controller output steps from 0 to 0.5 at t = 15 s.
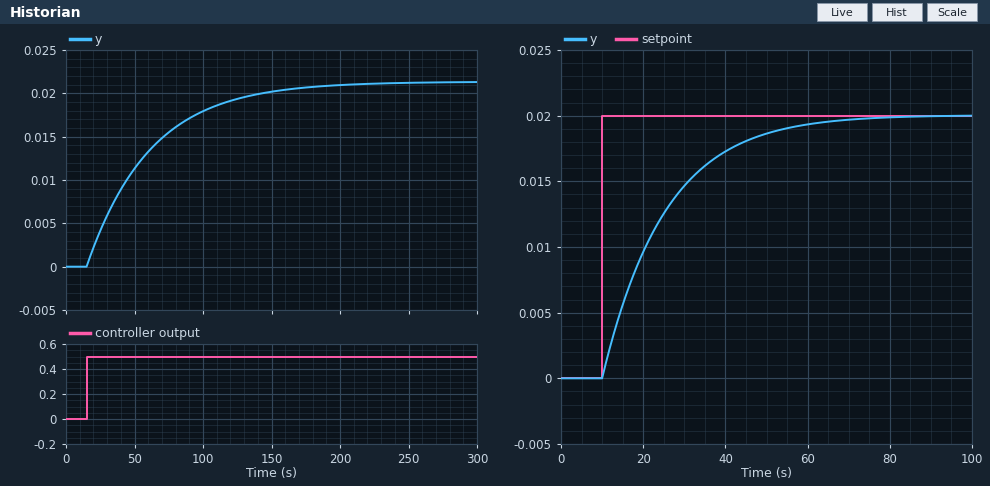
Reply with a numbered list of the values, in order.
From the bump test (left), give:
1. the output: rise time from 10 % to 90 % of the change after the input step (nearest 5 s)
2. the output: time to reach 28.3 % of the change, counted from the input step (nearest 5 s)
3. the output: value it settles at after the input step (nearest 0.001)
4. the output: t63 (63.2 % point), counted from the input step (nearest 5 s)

1. 100 s
2. 15 s
3. 0.021
4. 45 s
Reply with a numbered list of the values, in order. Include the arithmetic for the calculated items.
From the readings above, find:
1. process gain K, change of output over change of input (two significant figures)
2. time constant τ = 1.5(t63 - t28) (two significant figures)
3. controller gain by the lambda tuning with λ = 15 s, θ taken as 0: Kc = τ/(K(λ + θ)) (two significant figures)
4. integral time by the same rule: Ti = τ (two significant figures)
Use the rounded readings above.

1. (0.021 - 0) / 0.5 = 0.042
2. 1.5 × (45 - 15) = 45 s
3. 45 / (0.042 × (15 + 0)) = 71
4. 45 s
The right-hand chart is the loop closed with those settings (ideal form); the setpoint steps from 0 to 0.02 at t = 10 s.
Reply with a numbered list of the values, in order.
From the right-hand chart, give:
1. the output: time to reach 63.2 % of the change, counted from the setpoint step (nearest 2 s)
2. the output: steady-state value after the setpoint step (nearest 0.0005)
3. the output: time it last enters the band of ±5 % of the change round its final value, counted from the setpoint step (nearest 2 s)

1. 16 s
2. 0.0200
3. 44 s
